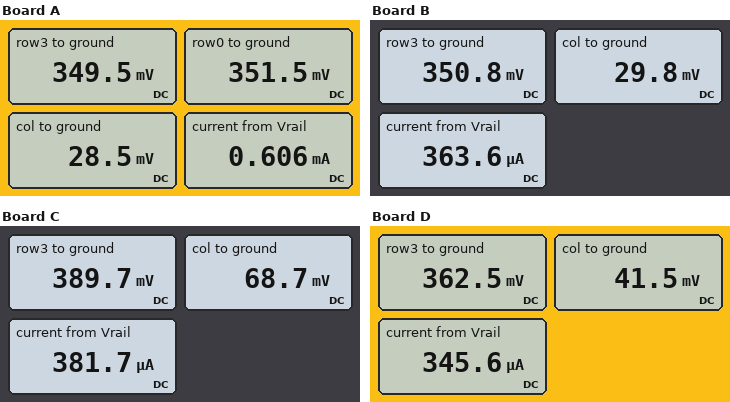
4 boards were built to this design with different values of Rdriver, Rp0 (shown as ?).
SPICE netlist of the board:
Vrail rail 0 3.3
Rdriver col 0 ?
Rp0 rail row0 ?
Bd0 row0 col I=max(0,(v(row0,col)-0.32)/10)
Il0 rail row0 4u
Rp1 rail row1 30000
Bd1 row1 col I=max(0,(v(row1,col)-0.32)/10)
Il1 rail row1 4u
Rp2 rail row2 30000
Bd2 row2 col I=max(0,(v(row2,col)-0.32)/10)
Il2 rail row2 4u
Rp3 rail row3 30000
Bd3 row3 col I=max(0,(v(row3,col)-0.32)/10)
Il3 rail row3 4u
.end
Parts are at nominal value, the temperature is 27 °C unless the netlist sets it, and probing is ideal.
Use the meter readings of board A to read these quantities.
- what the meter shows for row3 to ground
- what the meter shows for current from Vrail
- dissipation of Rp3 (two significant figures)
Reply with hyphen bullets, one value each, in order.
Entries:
- 349.5 mV
- 0.606 mA
- 290 µW
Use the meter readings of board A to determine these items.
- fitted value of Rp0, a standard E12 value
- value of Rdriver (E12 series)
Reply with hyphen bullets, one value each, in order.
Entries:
- 10 kΩ
- 47 Ω
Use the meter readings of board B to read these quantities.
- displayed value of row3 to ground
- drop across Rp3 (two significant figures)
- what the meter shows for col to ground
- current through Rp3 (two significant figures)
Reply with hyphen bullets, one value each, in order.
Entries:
- 350.8 mV
- 2.9 V
- 29.8 mV
- 98 µA
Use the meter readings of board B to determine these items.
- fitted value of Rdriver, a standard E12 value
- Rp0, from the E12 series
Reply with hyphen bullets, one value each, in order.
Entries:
- 82 Ω
- 56 kΩ
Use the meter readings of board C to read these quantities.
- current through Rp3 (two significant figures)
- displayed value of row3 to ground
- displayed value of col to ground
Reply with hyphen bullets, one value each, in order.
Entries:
- 97 µA
- 389.7 mV
- 68.7 mV
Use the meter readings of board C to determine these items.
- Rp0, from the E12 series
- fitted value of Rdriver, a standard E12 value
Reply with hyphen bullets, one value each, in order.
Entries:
- 39 kΩ
- 180 Ω
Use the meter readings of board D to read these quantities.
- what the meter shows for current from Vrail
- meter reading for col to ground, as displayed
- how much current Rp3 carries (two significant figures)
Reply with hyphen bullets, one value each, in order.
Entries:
- 345.6 µA
- 41.5 mV
- 98 µA
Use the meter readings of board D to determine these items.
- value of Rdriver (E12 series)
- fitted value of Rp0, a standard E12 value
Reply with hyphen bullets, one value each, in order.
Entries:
- 120 Ω
- 82 kΩ
